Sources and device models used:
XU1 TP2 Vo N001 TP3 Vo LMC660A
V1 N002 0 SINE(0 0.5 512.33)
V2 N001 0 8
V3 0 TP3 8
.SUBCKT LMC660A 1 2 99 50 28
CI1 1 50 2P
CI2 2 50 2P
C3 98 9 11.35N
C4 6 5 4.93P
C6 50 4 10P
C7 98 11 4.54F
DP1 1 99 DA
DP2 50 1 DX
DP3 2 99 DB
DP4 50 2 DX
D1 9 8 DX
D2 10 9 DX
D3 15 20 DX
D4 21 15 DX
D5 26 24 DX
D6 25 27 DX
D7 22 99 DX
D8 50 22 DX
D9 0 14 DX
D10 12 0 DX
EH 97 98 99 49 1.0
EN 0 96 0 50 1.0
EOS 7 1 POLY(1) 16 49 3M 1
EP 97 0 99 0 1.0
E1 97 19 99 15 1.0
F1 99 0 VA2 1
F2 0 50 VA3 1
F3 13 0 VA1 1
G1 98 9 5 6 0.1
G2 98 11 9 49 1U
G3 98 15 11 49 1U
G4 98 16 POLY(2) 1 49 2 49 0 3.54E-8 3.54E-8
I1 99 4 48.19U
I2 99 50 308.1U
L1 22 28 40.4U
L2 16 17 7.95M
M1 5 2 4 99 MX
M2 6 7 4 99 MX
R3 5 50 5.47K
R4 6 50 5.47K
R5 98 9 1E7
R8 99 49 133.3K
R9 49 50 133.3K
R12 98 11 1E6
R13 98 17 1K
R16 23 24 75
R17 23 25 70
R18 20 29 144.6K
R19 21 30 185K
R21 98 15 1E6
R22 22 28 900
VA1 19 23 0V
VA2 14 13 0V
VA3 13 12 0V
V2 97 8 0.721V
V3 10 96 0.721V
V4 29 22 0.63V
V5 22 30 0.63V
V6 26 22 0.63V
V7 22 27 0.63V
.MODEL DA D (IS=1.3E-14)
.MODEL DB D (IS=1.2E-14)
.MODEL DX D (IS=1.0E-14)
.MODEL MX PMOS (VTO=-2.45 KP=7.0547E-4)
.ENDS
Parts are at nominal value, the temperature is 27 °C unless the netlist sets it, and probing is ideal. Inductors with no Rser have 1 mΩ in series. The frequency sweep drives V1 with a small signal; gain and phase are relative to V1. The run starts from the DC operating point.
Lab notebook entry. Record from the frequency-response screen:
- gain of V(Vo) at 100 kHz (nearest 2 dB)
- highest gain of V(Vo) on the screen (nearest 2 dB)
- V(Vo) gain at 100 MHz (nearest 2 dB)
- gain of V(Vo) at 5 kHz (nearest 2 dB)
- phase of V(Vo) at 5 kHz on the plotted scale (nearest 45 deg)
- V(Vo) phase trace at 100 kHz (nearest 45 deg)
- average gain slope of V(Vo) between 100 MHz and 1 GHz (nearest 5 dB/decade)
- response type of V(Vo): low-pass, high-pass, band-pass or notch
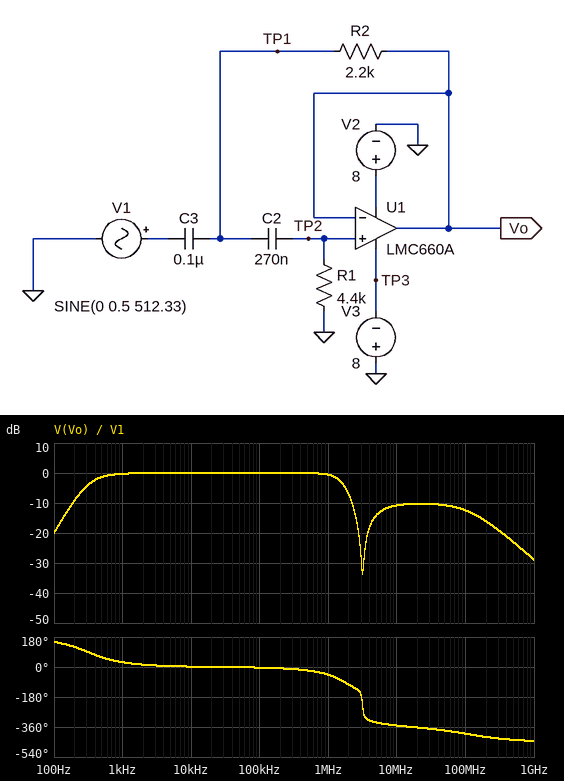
0 dB
0 dB
-12 dB
0 dB
0 deg
0 deg
-15 dB/decade
band-pass
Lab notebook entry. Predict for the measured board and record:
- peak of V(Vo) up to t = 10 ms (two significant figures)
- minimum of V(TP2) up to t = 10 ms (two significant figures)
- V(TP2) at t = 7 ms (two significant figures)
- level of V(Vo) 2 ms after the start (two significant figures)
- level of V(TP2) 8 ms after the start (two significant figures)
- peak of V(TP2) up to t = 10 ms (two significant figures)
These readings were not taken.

450 mV
-430 mV
-430 mV
420 mV
430 mV
450 mV
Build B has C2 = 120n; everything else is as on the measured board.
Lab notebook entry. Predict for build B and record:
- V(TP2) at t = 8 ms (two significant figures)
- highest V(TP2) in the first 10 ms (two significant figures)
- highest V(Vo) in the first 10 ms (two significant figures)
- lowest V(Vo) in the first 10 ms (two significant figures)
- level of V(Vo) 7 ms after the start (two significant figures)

340 mV
380 mV
390 mV
-380 mV
-350 mV
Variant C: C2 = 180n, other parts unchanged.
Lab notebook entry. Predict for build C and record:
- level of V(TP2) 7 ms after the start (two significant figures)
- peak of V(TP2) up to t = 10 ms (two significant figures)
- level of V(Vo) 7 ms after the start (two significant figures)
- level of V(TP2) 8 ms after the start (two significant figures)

-420 mV
430 mV
-410 mV
410 mV
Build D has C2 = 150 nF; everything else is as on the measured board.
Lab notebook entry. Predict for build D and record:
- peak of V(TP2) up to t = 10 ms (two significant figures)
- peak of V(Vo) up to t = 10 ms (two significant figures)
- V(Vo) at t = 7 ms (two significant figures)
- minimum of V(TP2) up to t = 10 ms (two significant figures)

410 mV
420 mV
-390 mV
-410 mV
